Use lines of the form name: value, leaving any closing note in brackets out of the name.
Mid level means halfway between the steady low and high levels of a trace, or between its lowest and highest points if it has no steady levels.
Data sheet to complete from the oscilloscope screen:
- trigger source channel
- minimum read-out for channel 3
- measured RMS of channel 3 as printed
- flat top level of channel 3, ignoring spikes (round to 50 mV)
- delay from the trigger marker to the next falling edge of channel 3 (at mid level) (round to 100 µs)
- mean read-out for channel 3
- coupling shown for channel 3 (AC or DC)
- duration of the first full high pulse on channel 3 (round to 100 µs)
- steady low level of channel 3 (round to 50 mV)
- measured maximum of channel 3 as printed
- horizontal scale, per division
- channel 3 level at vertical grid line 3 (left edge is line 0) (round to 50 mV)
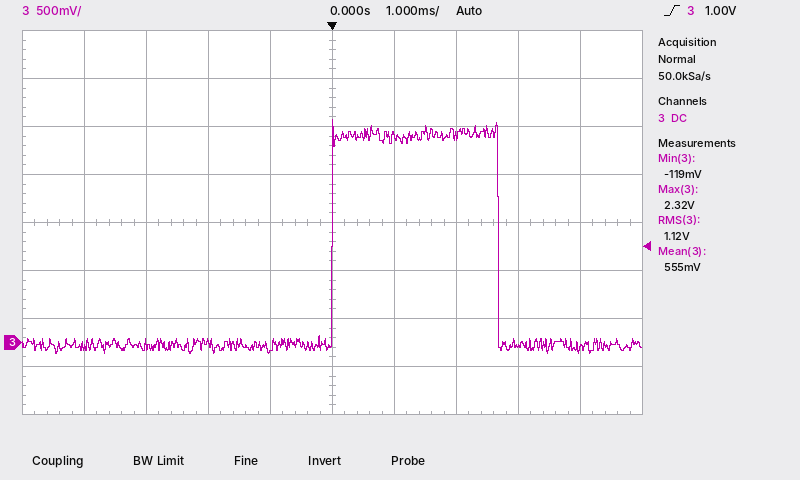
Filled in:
trigger source channel: channel 3
minimum read-out for channel 3: -119 mV
measured RMS of channel 3 as printed: 1.12 V
flat top level of channel 3, ignoring spikes: 2.15 V
delay from the trigger marker to the next falling edge of channel 3 (at mid level): 2.7 ms
mean read-out for channel 3: 555 mV
coupling shown for channel 3: DC
duration of the first full high pulse on channel 3: 2.7 ms
steady low level of channel 3: -50 mV
measured maximum of channel 3 as printed: 2.32 V
horizontal scale, per division: 1 ms
channel 3 level at vertical grid line 3 (left edge is line 0): 0 mV
